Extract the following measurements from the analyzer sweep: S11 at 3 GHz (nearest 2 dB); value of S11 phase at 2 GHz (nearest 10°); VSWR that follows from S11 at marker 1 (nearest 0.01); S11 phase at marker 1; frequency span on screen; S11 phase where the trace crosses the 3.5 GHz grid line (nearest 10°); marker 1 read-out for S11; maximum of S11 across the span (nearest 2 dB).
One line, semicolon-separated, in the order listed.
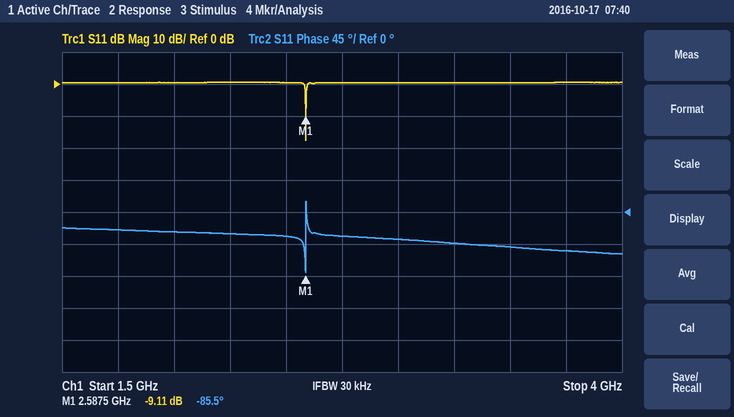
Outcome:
0 dB; -30°; 2.08; -85.5°; 2.5 GHz; -50°; -9.11 dB; 0 dB
